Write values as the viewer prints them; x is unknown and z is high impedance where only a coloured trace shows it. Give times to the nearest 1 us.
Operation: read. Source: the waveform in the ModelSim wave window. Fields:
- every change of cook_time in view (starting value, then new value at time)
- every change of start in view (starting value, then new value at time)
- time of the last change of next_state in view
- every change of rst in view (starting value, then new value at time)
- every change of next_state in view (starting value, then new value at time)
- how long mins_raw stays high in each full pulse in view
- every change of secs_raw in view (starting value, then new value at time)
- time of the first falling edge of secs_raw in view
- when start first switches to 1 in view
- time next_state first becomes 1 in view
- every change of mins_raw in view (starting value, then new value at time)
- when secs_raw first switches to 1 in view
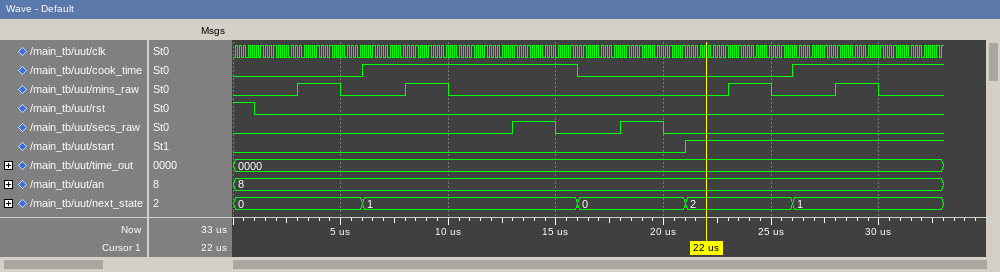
0, 1 at 6 us, 0 at 16 us, 1 at 26 us
0, 1 at 21 us
26 us
1, 0 at 1 us
0, 1 at 6 us, 0 at 16 us, 2 at 21 us, 1 at 26 us
2 us, 2 us, 2 us, 2 us
0, 1 at 13 us, 0 at 15 us, 1 at 18 us, 0 at 20 us
15 us
21 us
6 us
0, 1 at 3 us, 0 at 5 us, 1 at 8 us, 0 at 10 us, 1 at 23 us, 0 at 25 us, 1 at 28 us, 0 at 30 us
13 us
